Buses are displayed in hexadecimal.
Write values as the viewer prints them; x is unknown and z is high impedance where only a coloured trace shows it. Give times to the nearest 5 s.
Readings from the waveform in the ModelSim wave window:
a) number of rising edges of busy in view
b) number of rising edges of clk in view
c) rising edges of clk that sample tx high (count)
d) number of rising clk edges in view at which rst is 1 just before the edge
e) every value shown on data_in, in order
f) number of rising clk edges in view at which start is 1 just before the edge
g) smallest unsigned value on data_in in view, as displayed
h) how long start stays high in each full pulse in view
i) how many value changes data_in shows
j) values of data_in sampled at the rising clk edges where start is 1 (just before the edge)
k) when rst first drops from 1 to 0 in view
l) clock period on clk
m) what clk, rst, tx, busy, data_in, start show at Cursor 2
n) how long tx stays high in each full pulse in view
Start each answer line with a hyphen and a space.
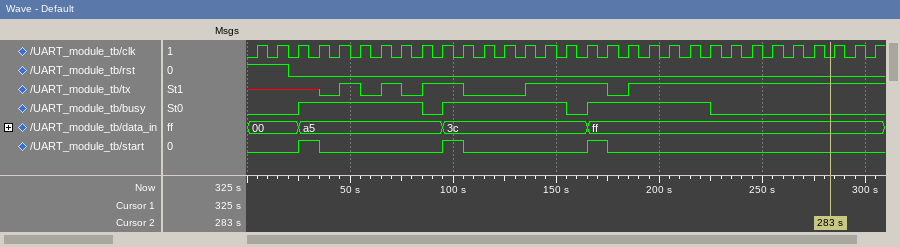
- 3
- 31
- 20
- 2
- 00, a5, 3c, ff
- 3
- 00
- 10 s, 10 s, 10 s
- 3
- a5, 3c, ff
- 20 s
- 10 s
- clk=0, rst=0, tx=1, busy=0, data_in=ff, start=0
- 10 s, 10 s, 20 s, 40 s
